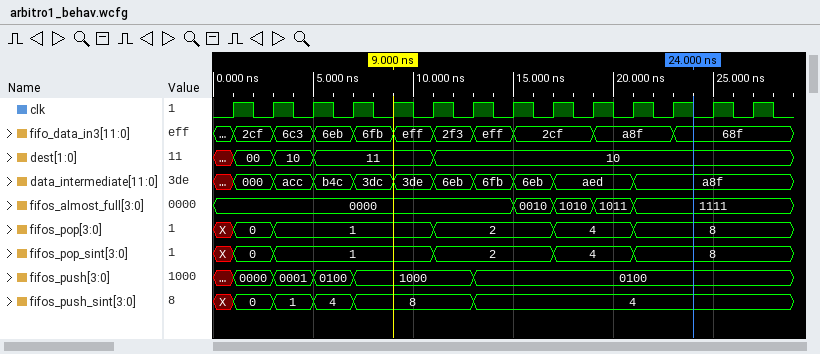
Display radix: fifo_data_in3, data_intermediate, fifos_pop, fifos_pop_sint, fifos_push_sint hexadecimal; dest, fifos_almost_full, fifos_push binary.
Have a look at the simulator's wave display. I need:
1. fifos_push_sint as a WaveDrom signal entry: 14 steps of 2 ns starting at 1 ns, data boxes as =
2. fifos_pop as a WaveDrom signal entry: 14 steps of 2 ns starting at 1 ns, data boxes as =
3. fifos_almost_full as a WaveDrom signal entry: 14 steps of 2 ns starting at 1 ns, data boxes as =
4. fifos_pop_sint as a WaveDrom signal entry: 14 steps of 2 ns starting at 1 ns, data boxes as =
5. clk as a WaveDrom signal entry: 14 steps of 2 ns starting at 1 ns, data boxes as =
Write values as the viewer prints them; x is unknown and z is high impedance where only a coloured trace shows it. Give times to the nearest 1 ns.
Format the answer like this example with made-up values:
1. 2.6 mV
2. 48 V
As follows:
1. {name: 'fifos_push_sint', wave: '====..=.......', data: '0 1 4 8 4'}
2. {name: 'fifos_pop', wave: '==...=..=.=...', data: '0 1 2 4 8'}
3. {name: 'fifos_almost_full', wave: '=......====...', data: '0000 0010 1010 1011 1111'}
4. {name: 'fifos_pop_sint', wave: '==...=..=.=...', data: '0 1 2 4 8'}
5. {name: 'clk', wave: 'p.............'}
